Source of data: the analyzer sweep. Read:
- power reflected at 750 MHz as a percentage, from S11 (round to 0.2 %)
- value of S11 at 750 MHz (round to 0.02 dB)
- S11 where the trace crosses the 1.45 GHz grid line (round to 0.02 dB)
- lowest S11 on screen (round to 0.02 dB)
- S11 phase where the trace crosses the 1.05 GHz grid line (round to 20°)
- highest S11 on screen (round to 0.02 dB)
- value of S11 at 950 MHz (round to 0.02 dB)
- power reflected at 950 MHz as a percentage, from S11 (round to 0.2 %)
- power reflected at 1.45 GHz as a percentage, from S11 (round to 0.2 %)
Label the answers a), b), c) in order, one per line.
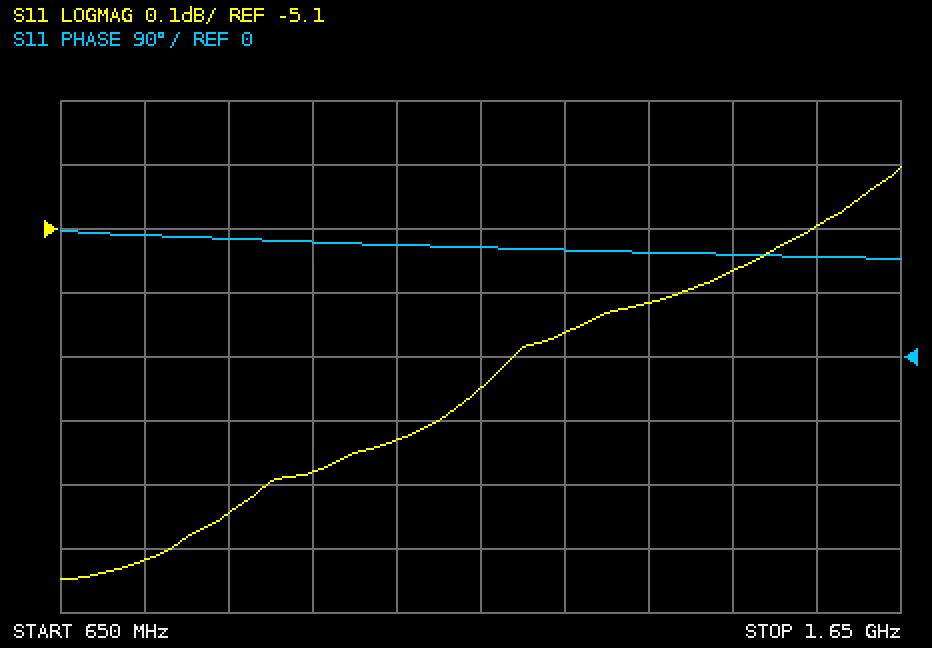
a) 27.4 %
b) -5.62 dB
c) -5.16 dB
d) -5.64 dB
e) 160°
f) -5.00 dB
g) -5.48 dB
h) 28.4 %
i) 30.4 %
